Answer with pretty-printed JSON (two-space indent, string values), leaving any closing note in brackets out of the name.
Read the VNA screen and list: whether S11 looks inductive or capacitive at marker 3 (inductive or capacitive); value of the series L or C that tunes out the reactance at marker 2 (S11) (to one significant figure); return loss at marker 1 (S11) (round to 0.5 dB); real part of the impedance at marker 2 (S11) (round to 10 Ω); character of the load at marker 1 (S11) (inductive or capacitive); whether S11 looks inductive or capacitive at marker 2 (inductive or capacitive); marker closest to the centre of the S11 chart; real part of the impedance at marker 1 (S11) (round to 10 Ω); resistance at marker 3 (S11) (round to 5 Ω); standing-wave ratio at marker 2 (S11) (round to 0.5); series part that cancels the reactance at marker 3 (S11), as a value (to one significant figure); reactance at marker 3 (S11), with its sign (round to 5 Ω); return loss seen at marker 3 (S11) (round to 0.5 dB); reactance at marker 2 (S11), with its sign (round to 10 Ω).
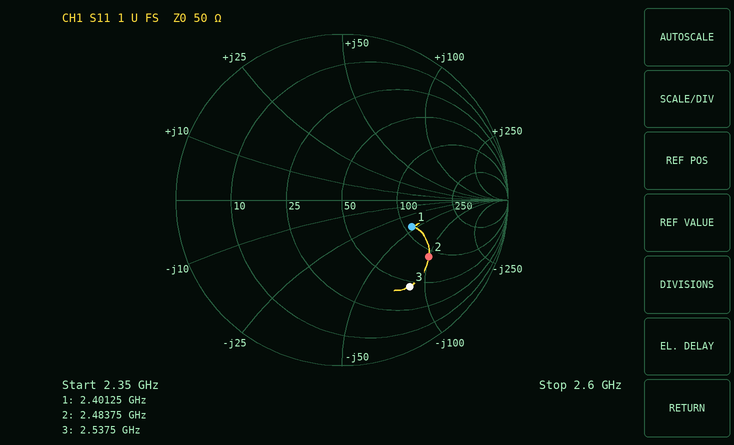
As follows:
{
  "whether S11 looks inductive or capacitive at marker 3": "capacitive",
  "value of the series L or C that tunes out the reactance at marker 2 (S11)": "6 nH",
  "return loss at marker 1 (S11)": "7.0 dB",
  "real part of the impedance at marker 2 (S11)": "90 Ω",
  "character of the load at marker 1 (S11)": "capacitive",
  "whether S11 looks inductive or capacitive at marker 2": "capacitive",
  "marker closest to the centre of the S11 chart": "marker 1",
  "real part of the impedance at marker 1 (S11)": "110 Ω",
  "resistance at marker 3 (S11)": "45 Ω",
  "standing-wave ratio at marker 2 (S11)": "4.5",
  "series part that cancels the reactance at marker 3 (S11), as a value": "5 nH",
  "reactance at marker 3 (S11), with its sign": "-85 Ω",
  "return loss seen at marker 3 (S11)": "3.5 dB",
  "reactance at marker 2 (S11), with its sign": "-100 Ω"
}
